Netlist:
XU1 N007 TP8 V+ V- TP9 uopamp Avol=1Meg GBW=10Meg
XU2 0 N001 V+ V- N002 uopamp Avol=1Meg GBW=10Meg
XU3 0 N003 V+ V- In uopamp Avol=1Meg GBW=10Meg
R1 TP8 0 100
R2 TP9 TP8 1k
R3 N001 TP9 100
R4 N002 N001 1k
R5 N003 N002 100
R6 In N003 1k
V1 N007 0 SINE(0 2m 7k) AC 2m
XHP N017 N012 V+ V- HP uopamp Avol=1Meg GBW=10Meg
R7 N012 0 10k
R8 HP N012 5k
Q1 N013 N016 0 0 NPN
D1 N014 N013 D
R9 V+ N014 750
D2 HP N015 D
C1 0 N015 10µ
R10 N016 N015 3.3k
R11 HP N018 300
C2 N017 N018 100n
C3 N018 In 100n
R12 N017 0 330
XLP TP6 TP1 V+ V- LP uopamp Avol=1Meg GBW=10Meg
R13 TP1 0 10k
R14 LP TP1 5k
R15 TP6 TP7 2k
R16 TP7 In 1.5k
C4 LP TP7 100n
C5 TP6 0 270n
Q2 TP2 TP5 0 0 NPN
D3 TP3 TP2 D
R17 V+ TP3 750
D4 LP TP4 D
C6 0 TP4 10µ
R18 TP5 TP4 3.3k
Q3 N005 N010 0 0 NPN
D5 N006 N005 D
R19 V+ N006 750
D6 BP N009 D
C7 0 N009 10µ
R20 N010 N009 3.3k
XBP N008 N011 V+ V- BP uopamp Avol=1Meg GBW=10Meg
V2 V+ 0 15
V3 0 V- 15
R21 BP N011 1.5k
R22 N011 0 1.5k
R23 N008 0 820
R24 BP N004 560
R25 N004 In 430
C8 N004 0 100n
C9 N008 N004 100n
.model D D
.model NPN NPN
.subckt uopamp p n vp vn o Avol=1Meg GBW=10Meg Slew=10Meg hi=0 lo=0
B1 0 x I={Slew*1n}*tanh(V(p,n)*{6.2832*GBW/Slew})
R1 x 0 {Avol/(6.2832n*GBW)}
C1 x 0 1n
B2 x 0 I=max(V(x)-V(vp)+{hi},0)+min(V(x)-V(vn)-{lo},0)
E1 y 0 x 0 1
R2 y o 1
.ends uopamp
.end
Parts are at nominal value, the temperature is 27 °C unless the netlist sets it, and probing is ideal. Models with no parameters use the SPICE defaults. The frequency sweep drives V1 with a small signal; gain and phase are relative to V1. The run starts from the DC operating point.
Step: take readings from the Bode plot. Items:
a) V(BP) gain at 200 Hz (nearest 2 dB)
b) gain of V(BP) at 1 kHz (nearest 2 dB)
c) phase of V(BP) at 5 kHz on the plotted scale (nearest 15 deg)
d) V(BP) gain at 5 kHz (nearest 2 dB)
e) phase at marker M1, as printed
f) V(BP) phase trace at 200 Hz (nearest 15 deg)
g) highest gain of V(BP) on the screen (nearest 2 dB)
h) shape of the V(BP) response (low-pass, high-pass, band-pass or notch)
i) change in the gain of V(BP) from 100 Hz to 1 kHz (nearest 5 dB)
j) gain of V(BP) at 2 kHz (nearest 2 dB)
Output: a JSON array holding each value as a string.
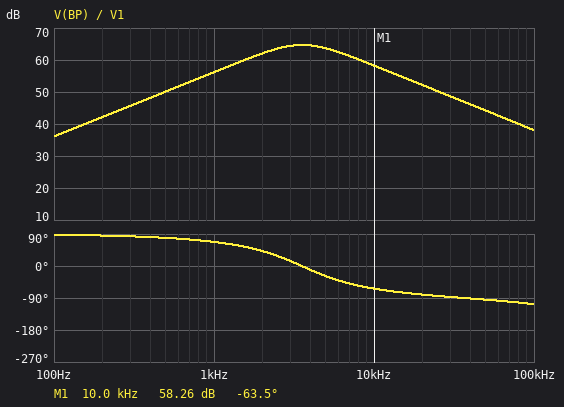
["42 dB", "56 dB", "-30 deg", "64 dB", "-63.5 deg", "90 deg", "64 dB", "band-pass", "20 dB", "62 dB"]
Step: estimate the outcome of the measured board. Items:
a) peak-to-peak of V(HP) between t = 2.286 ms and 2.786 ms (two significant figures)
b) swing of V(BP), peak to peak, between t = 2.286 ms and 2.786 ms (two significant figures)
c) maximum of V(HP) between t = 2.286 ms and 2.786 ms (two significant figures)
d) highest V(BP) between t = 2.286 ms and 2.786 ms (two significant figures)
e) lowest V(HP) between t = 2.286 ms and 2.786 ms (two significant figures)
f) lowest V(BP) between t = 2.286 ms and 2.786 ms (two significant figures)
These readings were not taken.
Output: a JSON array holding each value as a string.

["6.0 V", "4.6 V", "3.0 V", "2.3 V", "-3.0 V", "-2.3 V"]
